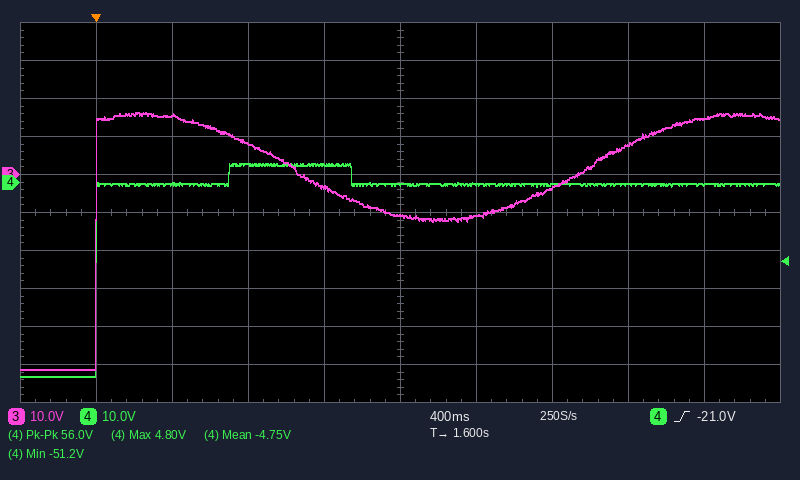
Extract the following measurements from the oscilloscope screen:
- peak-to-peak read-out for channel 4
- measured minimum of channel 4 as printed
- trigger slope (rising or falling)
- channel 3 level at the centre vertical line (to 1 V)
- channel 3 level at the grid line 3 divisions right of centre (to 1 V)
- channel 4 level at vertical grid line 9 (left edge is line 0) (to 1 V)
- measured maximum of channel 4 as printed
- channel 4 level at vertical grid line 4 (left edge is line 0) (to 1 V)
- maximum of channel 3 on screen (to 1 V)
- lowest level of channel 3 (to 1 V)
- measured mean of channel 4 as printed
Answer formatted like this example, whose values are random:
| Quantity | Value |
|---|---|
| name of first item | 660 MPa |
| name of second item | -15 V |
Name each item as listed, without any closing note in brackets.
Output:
| Quantity | Value |
|---|---|
| peak-to-peak read-out for channel 4 | 56.0 V |
| measured minimum of channel 4 as printed | -51.2 V |
| trigger slope | rising |
| channel 3 level at the centre vertical line | -11 V |
| channel 3 level at the grid line 3 divisions right of centre | 8 V |
| channel 4 level at vertical grid line 9 (left edge is line 0) | -1 V |
| measured maximum of channel 4 as printed | 4.80 V |
| channel 4 level at vertical grid line 4 (left edge is line 0) | 5 V |
| maximum of channel 3 on screen | 16 V |
| lowest level of channel 3 | -51 V |
| measured mean of channel 4 as printed | -4.75 V |
